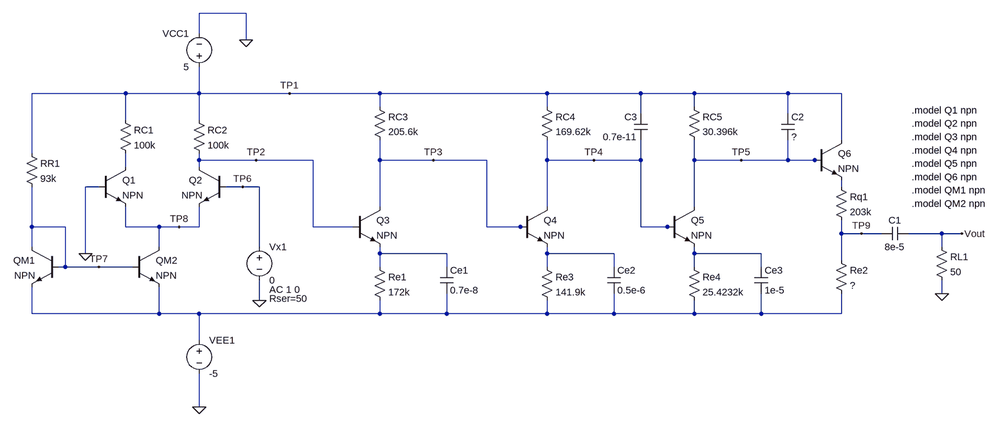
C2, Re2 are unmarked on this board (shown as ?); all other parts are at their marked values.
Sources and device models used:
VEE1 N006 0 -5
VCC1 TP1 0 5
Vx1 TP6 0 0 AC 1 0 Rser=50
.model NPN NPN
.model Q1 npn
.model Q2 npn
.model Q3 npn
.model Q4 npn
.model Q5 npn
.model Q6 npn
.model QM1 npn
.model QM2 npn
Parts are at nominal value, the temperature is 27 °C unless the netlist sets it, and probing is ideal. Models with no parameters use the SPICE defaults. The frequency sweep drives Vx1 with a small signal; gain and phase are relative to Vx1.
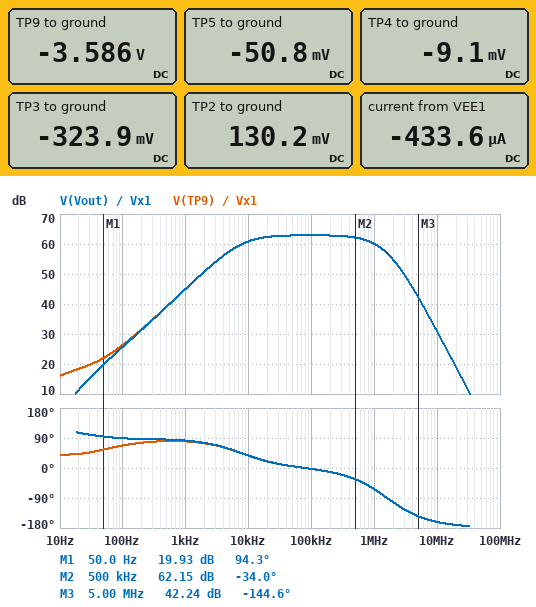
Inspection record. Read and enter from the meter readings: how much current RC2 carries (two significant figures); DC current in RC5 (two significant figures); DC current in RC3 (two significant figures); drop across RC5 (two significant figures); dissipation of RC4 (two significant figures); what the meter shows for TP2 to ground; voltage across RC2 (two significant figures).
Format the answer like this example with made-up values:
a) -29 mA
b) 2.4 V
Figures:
a) 49 µA
b) 170 µA
c) 26 µA
d) 5.1 V
e) 150 µW
f) 130.2 mV
g) 4.9 V
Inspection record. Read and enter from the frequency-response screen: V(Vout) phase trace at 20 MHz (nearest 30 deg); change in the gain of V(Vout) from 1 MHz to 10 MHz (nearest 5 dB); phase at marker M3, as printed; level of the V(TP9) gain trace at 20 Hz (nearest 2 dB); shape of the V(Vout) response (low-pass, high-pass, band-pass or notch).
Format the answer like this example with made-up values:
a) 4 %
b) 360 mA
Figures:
a) -180 deg
b) -30 dB
c) -144.6 deg
d) 18 dB
e) band-pass
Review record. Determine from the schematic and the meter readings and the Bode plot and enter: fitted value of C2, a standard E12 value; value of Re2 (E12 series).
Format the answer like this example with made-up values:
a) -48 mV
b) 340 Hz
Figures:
a) 3.3 pF
b) 100 kΩ
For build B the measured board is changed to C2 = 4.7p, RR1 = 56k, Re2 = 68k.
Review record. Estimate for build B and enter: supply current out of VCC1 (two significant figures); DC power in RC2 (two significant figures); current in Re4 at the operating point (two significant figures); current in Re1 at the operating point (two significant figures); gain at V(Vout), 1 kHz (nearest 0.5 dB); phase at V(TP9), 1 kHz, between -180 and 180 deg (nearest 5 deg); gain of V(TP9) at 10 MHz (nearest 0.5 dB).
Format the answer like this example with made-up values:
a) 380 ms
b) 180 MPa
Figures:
a) 500 µA
b) 320 µW
c) 150 µA
d) 21 µA
e) -49.0 dB
f) 85 deg
g) -43.5 dB
